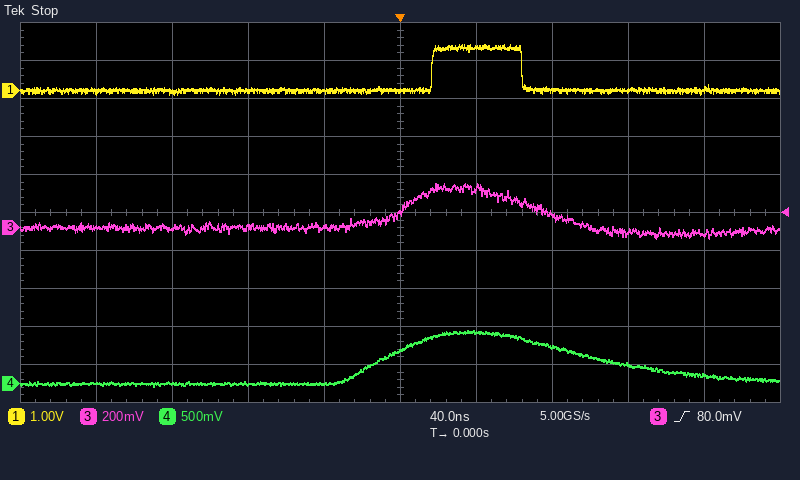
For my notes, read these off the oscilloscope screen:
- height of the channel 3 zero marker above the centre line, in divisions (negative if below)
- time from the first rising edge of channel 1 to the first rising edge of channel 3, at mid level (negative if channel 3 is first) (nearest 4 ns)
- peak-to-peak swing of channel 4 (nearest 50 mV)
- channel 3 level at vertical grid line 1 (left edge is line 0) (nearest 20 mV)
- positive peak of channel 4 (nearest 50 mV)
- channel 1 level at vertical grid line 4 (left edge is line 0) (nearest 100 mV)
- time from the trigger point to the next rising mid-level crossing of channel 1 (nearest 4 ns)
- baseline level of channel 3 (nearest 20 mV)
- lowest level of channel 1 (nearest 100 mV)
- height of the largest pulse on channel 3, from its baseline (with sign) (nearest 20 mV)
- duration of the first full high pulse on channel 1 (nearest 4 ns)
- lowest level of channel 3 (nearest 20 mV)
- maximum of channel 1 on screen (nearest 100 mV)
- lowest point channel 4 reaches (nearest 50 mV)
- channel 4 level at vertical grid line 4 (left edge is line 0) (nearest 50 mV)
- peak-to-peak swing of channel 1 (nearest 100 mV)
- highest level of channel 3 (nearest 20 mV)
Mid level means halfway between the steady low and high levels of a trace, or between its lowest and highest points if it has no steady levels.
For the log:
-0.4 div
-16 ns
750 mV
0 mV
700 mV
0.0 V
16 ns
0 mV
-100 mV
+240 mV
48 ns
-60 mV
1.2 V
-50 mV
0 mV
1.3 V
240 mV
